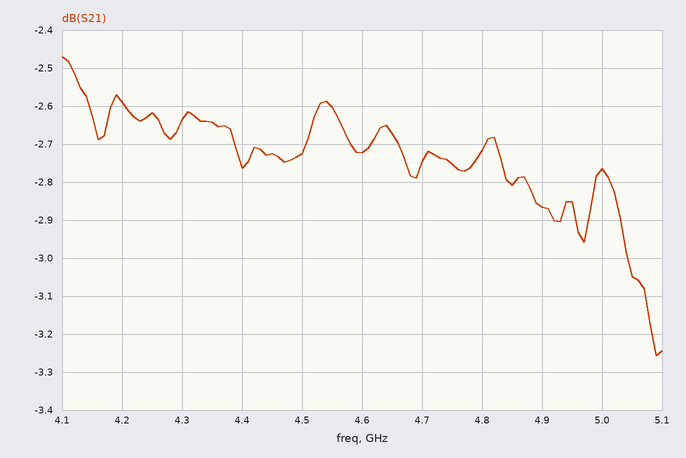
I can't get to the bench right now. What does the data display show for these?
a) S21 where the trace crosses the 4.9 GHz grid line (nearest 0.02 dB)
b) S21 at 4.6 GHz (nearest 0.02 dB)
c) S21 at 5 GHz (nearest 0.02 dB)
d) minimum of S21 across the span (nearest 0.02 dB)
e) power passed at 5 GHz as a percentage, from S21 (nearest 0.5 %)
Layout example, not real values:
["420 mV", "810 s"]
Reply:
["-2.86 dB", "-2.72 dB", "-2.76 dB", "-3.26 dB", "53.0 %"]
